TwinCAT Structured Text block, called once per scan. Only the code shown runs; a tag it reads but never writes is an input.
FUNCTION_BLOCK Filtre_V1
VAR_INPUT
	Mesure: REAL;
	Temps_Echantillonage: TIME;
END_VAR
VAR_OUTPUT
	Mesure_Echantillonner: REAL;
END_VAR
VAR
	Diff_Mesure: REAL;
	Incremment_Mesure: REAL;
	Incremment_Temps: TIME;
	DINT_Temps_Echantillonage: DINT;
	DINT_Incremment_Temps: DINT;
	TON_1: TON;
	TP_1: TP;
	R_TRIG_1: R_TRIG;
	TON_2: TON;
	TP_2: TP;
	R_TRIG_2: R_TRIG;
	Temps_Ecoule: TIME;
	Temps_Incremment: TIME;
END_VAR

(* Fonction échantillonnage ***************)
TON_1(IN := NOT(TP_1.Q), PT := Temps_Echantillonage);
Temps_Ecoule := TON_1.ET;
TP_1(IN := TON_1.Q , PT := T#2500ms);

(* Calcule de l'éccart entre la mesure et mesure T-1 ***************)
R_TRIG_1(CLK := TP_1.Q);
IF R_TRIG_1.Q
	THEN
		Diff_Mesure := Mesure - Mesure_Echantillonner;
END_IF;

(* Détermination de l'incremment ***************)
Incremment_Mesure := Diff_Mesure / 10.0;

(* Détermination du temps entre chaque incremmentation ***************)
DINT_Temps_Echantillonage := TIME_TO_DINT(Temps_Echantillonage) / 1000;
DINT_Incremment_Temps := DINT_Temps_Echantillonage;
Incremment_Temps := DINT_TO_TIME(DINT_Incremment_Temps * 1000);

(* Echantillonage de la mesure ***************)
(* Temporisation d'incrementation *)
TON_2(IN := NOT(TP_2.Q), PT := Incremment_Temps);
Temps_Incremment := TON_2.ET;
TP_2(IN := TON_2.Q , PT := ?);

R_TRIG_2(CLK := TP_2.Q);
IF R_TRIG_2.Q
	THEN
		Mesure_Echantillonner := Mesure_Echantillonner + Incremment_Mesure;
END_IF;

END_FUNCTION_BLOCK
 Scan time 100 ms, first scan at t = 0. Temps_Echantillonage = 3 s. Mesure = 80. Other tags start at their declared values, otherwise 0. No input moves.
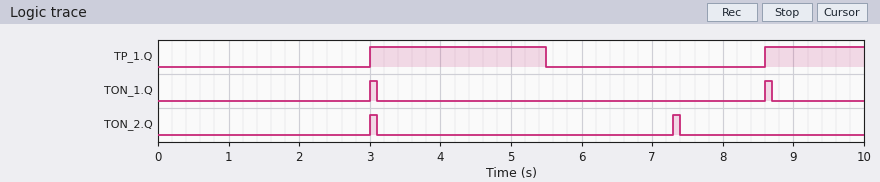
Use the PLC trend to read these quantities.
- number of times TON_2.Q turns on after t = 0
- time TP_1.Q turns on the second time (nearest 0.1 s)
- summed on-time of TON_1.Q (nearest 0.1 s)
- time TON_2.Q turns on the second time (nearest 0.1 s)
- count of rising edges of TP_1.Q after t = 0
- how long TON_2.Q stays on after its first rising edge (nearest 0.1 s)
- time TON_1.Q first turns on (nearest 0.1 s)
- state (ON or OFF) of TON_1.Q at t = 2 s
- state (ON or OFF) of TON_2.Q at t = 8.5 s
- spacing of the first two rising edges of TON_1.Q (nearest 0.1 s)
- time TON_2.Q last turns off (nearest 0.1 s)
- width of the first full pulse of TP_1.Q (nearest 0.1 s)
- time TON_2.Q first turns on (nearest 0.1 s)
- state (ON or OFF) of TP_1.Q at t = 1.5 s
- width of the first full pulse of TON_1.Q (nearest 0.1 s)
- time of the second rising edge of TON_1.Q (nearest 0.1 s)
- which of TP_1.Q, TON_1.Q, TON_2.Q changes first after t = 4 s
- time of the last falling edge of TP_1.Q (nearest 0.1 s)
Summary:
2
8.6 s
0.2 s
7.3 s
2
0.1 s
3.0 s
OFF
OFF
5.6 s
7.4 s
2.5 s
3.0 s
OFF
0.1 s
8.6 s
TP_1.Q
5.5 s
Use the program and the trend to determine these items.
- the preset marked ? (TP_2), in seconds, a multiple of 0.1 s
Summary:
1.2 s
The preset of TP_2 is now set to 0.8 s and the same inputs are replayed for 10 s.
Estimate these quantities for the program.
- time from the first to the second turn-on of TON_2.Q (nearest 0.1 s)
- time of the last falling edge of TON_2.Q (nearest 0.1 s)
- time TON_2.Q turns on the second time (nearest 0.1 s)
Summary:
3.9 s
7.0 s
6.9 s
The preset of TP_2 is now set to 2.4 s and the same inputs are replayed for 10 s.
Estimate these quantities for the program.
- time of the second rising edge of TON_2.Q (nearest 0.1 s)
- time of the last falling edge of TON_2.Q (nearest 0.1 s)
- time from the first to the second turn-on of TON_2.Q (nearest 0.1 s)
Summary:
8.5 s
8.6 s
5.5 s
